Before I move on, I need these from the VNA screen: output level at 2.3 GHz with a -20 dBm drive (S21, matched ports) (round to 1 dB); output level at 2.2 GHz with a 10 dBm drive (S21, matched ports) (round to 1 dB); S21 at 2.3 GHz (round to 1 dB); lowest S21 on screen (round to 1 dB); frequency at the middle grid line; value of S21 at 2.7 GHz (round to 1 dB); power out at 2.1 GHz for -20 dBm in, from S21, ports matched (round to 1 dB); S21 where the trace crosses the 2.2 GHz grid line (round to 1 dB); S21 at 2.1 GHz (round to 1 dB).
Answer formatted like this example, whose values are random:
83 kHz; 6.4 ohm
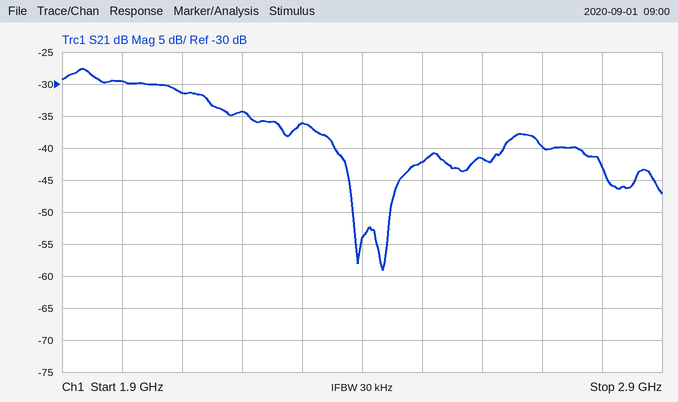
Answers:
-56 dBm; -24 dBm; -36 dB; -59 dB; 2.4 GHz; -40 dB; -51 dBm; -34 dB; -31 dB
